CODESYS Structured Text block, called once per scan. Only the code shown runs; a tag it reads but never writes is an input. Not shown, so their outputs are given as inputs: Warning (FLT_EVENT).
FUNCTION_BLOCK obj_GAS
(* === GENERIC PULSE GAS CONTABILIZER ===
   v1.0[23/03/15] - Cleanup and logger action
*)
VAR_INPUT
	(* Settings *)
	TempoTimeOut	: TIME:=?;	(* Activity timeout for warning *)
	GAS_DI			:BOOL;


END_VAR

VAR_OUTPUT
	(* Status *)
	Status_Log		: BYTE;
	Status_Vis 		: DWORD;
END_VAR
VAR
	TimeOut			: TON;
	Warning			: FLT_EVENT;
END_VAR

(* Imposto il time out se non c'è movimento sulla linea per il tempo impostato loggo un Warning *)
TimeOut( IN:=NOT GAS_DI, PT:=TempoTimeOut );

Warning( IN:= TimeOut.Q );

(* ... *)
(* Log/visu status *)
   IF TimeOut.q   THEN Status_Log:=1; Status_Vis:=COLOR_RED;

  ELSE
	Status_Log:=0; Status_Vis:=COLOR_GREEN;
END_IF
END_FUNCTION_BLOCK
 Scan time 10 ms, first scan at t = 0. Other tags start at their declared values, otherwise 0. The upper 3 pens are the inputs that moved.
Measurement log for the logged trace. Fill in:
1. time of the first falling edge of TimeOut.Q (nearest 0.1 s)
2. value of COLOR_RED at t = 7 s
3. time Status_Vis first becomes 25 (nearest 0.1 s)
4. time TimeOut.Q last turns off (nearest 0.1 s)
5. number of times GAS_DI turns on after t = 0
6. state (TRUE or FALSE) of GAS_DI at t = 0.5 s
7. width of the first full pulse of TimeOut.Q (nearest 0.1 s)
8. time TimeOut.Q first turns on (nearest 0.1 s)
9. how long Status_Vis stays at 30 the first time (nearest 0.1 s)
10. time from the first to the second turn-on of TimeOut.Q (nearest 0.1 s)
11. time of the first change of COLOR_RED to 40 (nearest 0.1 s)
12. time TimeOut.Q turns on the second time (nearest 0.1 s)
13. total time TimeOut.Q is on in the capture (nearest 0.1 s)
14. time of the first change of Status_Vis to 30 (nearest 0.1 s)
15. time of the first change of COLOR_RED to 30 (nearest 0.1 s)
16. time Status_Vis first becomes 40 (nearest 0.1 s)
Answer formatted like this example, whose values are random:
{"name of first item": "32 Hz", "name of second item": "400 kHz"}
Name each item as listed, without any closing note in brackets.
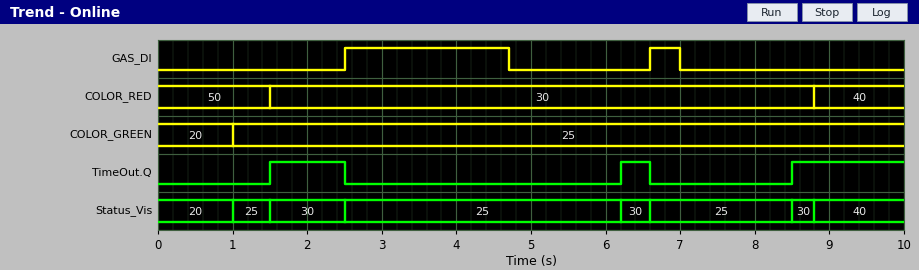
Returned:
{"time of the first falling edge of TimeOut.Q": "2.5 s", "value of COLOR_RED at t = 7 s": "30", "time Status_Vis first becomes 25": "1.0 s", "time TimeOut.Q last turns off": "6.6 s", "number of times GAS_DI turns on after t = 0": "2", "state (TRUE or FALSE) of GAS_DI at t = 0.5 s": "FALSE", "width of the first full pulse of TimeOut.Q": "1.0 s", "time TimeOut.Q first turns on": "1.5 s", "how long Status_Vis stays at 30 the first time": "1.0 s", "time from the first to the second turn-on of TimeOut.Q": "4.7 s", "time of the first change of COLOR_RED to 40": "8.8 s", "time TimeOut.Q turns on the second time": "6.2 s", "total time TimeOut.Q is on in the capture": "2.9 s", "time of the first change of Status_Vis to 30": "1.5 s", "time of the first change of COLOR_RED to 30": "1.5 s", "time Status_Vis first becomes 40": "8.8 s"}
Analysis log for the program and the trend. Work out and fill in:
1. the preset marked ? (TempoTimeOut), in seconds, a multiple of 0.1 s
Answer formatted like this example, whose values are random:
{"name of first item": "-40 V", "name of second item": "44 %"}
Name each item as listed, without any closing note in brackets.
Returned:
{"the preset marked ? (TempoTimeOut), in seconds, a multiple of 0.1 s": "1.5 s"}
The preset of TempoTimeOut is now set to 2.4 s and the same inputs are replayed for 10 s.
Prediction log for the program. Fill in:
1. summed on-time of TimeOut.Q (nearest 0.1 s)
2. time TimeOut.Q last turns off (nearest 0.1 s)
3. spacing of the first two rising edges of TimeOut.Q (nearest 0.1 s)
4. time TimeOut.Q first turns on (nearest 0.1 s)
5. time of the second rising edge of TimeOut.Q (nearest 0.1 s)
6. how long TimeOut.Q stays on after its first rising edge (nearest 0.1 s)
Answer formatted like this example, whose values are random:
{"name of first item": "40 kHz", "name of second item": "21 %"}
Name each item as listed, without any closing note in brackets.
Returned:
{"summed on-time of TimeOut.Q": "0.7 s", "time TimeOut.Q last turns off": "2.5 s", "spacing of the first two rising edges of TimeOut.Q": "7.0 s", "time TimeOut.Q first turns on": "2.4 s", "time of the second rising edge of TimeOut.Q": "9.4 s", "how long TimeOut.Q stays on after its first rising edge": "0.1 s"}
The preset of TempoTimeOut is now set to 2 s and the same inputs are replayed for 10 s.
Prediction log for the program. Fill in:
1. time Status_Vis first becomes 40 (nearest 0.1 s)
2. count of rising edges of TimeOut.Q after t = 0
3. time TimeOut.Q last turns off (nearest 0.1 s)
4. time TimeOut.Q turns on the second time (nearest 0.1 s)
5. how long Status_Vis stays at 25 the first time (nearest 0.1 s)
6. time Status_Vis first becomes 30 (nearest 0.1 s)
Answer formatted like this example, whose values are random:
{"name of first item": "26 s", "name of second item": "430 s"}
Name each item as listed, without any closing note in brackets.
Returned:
{"time Status_Vis first becomes 40": "9.0 s", "count of rising edges of TimeOut.Q after t = 0": "2", "time TimeOut.Q last turns off": "2.5 s", "time TimeOut.Q turns on the second time": "9.0 s", "how long Status_Vis stays at 25 the first time": "1.0 s", "time Status_Vis first becomes 30": "2.0 s"}
